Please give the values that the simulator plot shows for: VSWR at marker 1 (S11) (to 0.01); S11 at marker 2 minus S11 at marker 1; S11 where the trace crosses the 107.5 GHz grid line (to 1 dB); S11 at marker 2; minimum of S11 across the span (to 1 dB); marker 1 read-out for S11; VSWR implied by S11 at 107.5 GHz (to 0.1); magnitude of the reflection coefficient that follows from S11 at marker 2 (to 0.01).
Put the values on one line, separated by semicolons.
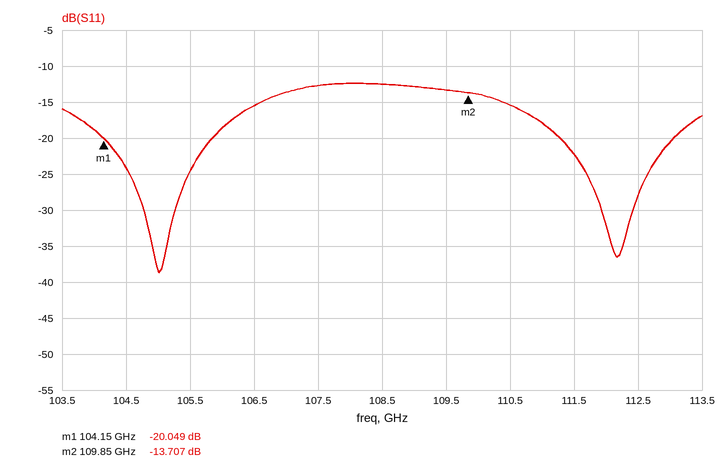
1.22; 6.342 dB; -13 dB; -13.707 dB; -39 dB; -20.049 dB; 1.6; 0.21
